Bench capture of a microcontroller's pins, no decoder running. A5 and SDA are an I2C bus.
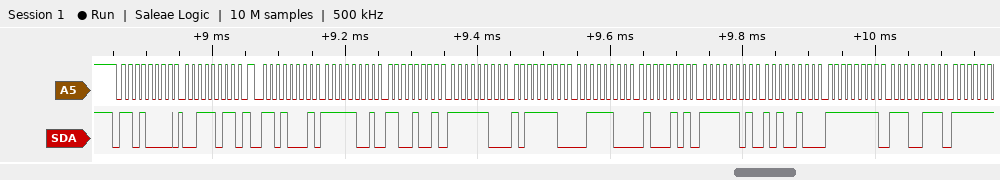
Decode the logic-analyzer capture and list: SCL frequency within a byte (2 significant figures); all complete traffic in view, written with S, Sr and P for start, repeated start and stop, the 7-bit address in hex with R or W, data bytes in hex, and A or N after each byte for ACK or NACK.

100 kHz
S 68W A 3B A Sr 68R A F9 A C9 A FC A BE A 3C A 45 A FD A A4 A FF A E7 A
